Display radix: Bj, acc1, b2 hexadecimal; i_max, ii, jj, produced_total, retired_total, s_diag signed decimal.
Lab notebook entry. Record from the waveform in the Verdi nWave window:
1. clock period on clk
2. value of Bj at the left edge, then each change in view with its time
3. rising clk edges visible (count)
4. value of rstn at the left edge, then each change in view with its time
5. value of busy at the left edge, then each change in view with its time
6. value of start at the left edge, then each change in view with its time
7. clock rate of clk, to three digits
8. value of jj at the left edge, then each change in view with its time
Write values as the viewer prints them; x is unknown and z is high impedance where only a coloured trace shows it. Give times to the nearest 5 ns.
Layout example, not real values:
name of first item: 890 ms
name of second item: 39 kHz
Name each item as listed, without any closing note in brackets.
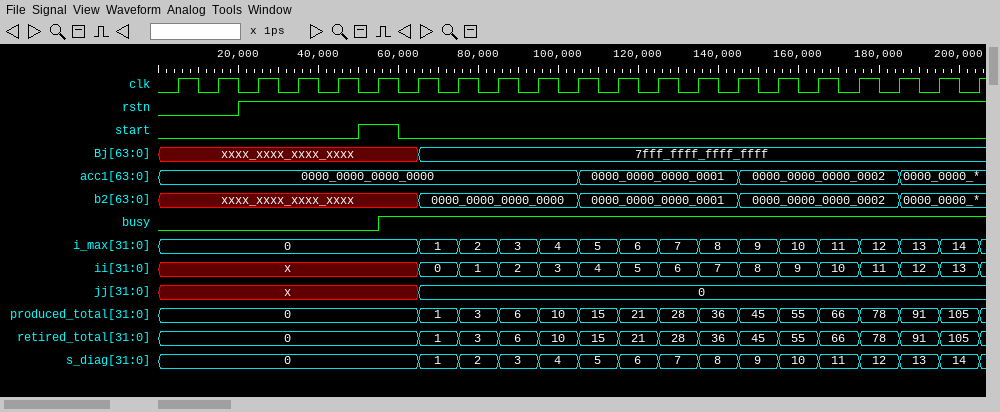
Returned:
clock period on clk: 10 ns
value of Bj at the left edge, then each change in view with its time: xxxx_xxxx_xxxx_xxxx, 7fff_ffff_ffff_ffff at 65 ns
rising clk edges visible: 21
value of rstn at the left edge, then each change in view with its time: 0, 1 at 20 ns
value of busy at the left edge, then each change in view with its time: 0, 1 at 55 ns
value of start at the left edge, then each change in view with its time: 0, 1 at 50 ns, 0 at 60 ns
clock rate of clk, to three digits: 100 MHz
value of jj at the left edge, then each change in view with its time: x, 0 at 65 ns
